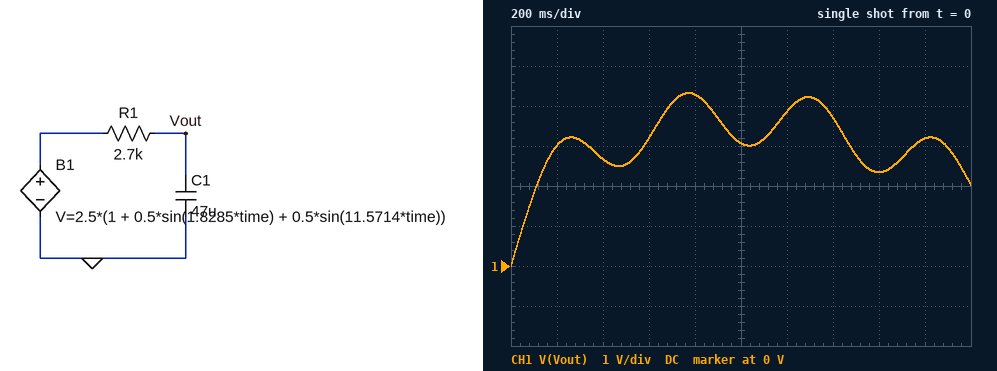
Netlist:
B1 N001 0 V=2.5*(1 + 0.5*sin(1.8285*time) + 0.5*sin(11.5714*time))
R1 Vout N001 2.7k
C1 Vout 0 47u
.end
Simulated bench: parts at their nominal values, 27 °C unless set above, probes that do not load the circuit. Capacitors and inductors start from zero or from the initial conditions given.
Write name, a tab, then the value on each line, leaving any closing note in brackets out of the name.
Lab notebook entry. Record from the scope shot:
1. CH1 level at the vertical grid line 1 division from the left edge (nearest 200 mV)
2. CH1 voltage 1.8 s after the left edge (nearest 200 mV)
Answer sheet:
CH1 level at the vertical grid line 1 division from the left edge	3.0 V
CH1 voltage 1.8 s after the left edge	3.2 V
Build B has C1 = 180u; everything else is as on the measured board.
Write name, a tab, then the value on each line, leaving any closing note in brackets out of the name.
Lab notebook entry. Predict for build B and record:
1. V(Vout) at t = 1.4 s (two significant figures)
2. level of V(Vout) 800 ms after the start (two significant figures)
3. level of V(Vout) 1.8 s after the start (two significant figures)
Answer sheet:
V(Vout) at t = 1.4 s	3.5 V
level of V(Vout) 800 ms after the start	3.0 V
level of V(Vout) 1.8 s after the start	3.1 V
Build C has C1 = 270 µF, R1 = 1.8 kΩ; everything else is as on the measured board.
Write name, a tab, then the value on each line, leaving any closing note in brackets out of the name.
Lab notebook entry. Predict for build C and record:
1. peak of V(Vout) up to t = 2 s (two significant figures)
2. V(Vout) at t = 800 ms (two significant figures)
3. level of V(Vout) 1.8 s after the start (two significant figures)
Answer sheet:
peak of V(Vout) up to t = 2 s	3.5 V
V(Vout) at t = 800 ms	3.0 V
level of V(Vout) 1.8 s after the start	3.1 V
